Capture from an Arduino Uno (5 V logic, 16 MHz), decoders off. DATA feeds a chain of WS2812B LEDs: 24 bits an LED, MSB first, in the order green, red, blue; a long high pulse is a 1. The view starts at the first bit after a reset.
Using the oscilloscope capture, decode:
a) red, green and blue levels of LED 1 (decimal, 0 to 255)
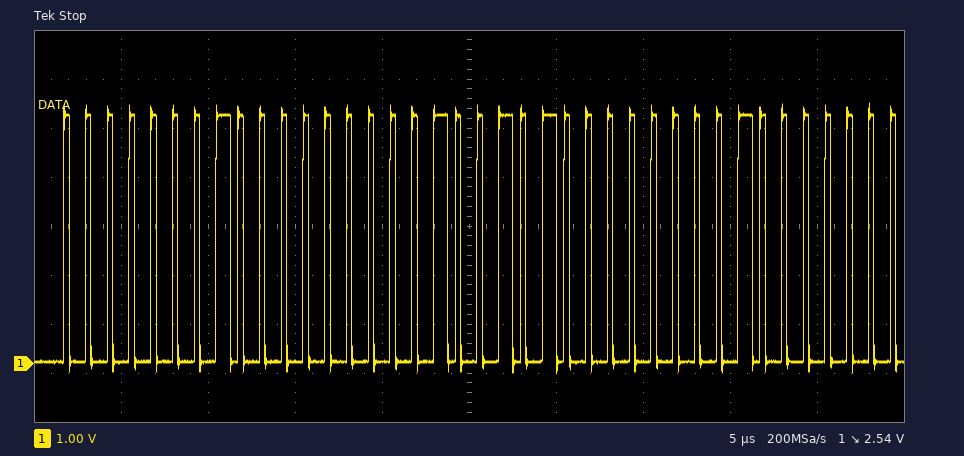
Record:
0, 1, 74
